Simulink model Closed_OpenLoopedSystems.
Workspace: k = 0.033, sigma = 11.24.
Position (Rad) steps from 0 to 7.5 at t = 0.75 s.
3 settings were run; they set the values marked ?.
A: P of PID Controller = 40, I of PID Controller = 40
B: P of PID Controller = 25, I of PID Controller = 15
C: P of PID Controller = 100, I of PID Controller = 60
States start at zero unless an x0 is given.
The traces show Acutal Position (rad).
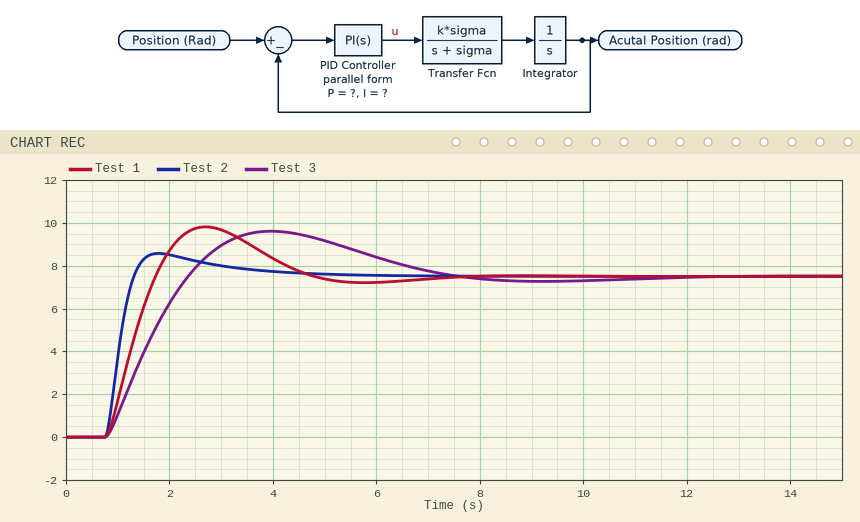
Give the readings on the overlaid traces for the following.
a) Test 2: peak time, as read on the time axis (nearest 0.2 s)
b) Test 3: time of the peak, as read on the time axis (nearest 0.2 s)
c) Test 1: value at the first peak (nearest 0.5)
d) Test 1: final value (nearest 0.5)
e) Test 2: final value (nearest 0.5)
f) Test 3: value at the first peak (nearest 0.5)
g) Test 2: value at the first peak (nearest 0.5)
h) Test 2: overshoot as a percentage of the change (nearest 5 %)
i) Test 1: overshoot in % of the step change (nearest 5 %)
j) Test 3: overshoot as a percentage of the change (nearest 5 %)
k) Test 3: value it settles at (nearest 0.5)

1.8 s
4.0 s
10.0
7.5
7.5
9.5
8.5
15 %
30 %
30 %
7.5
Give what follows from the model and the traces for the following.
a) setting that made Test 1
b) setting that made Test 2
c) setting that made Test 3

A
C
B
